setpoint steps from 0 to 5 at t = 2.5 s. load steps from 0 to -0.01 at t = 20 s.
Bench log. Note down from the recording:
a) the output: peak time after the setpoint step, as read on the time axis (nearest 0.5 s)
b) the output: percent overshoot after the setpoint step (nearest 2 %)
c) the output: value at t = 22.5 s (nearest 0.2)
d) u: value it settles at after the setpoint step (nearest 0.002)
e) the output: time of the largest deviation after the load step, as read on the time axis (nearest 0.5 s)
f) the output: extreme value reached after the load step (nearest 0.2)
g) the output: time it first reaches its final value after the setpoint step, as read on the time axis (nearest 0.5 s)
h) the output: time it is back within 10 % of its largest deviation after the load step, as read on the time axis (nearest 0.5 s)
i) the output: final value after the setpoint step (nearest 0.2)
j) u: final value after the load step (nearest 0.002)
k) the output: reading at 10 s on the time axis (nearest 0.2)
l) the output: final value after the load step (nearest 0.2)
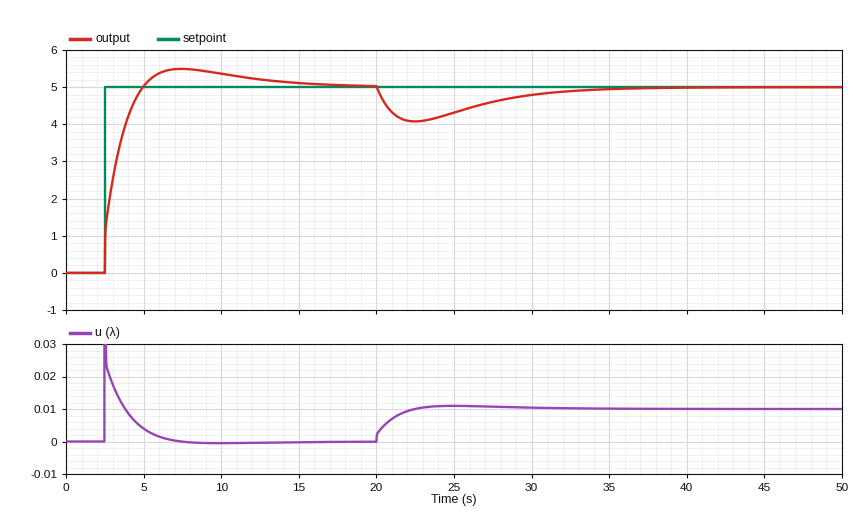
7.5 s
10 %
4.0
0.000
22.5 s
4.0
5.0 s
33.0 s
5.0
0.010
5.4
5.0
